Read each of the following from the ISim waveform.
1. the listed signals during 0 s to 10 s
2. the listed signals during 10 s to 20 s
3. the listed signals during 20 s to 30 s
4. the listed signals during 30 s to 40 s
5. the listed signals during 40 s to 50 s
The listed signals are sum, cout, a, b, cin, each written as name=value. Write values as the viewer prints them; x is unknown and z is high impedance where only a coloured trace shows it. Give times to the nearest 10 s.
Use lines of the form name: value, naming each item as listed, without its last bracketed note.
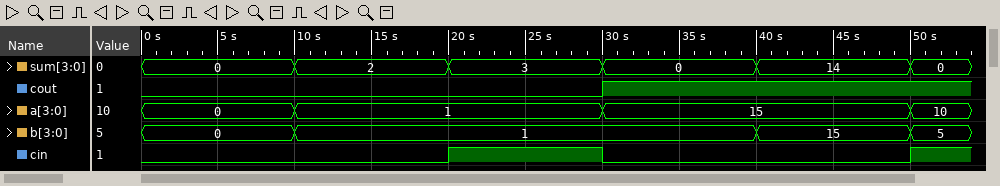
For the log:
the listed signals during 0 s to 10 s: sum=0, cout=0, a=0, b=0, cin=0
the listed signals during 10 s to 20 s: sum=2, cout=0, a=1, b=1, cin=0
the listed signals during 20 s to 30 s: sum=3, cout=0, a=1, b=1, cin=1
the listed signals during 30 s to 40 s: sum=0, cout=1, a=15, b=1, cin=0
the listed signals during 40 s to 50 s: sum=14, cout=1, a=15, b=15, cin=0
